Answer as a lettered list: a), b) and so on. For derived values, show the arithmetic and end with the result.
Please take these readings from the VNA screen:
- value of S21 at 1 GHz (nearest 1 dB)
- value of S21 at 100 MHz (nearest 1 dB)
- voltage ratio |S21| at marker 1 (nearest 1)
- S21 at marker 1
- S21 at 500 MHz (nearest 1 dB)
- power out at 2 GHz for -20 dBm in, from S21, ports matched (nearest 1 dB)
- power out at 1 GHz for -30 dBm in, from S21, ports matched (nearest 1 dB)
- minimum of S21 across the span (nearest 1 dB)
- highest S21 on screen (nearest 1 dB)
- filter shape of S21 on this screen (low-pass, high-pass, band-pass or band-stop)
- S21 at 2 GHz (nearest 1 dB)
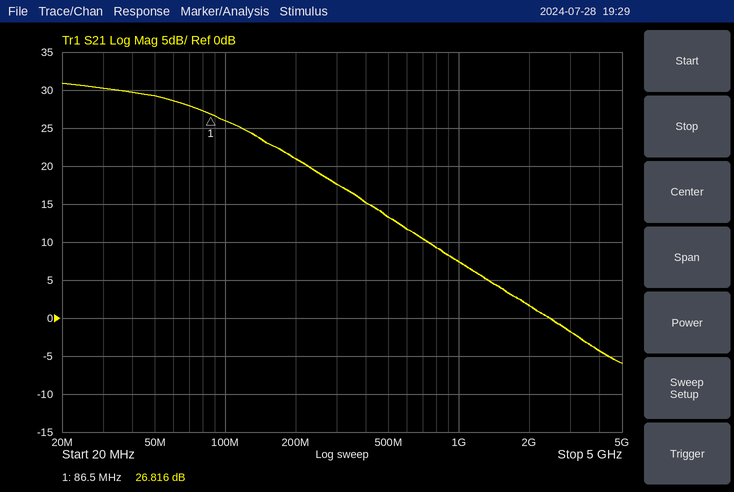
a) 7 dB
b) 26 dB
c) 10^(26.816/20) ≈ 22
d) 26.816 dB
e) 13 dB
f) -20 dBm + (2 dB) = -18 dBm
g) -30 dBm + (7 dB) = -23 dBm
h) -6 dB
i) 31 dB
j) low-pass
k) 2 dB
